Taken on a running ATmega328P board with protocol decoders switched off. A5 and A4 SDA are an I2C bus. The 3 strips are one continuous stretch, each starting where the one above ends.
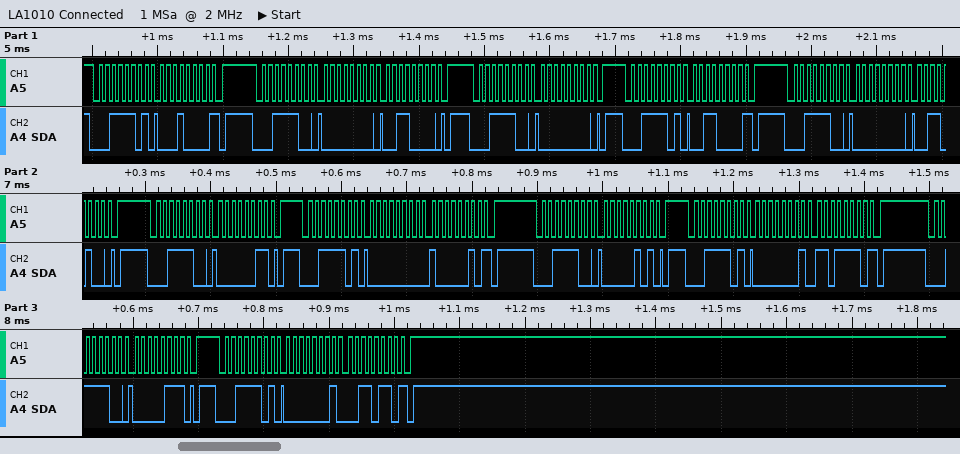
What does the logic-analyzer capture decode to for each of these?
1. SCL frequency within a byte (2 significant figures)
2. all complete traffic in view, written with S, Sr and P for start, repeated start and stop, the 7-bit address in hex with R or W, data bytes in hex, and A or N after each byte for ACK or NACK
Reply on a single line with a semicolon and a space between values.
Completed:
100 kHz; S 1ER A 10 N P S 1EW A 00 A 30 A P S 1EW A 00 A P S 1ER A 30 N P S 1EW A 00 A 34 A P S 1EW A 03 A P S 1ER A 00 A 82 N P S 1EW A 05 A P S 1ER A 01 A DE N P S 1EW A 07 A P S 1ER A 01 A 36 N P
